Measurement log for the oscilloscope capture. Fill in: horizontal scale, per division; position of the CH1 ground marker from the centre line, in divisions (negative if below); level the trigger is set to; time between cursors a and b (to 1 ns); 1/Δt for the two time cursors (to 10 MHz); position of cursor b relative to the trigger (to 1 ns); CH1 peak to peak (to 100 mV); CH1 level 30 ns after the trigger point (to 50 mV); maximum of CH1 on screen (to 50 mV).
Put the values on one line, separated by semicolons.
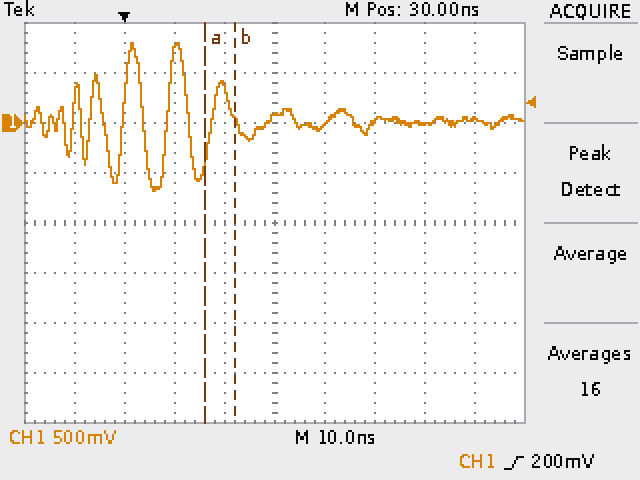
10 ns; +2.0 div; 200 mV; 6 ns; 170 MHz; +22 ns; 1.50 V; 50 mV; 800 mV
